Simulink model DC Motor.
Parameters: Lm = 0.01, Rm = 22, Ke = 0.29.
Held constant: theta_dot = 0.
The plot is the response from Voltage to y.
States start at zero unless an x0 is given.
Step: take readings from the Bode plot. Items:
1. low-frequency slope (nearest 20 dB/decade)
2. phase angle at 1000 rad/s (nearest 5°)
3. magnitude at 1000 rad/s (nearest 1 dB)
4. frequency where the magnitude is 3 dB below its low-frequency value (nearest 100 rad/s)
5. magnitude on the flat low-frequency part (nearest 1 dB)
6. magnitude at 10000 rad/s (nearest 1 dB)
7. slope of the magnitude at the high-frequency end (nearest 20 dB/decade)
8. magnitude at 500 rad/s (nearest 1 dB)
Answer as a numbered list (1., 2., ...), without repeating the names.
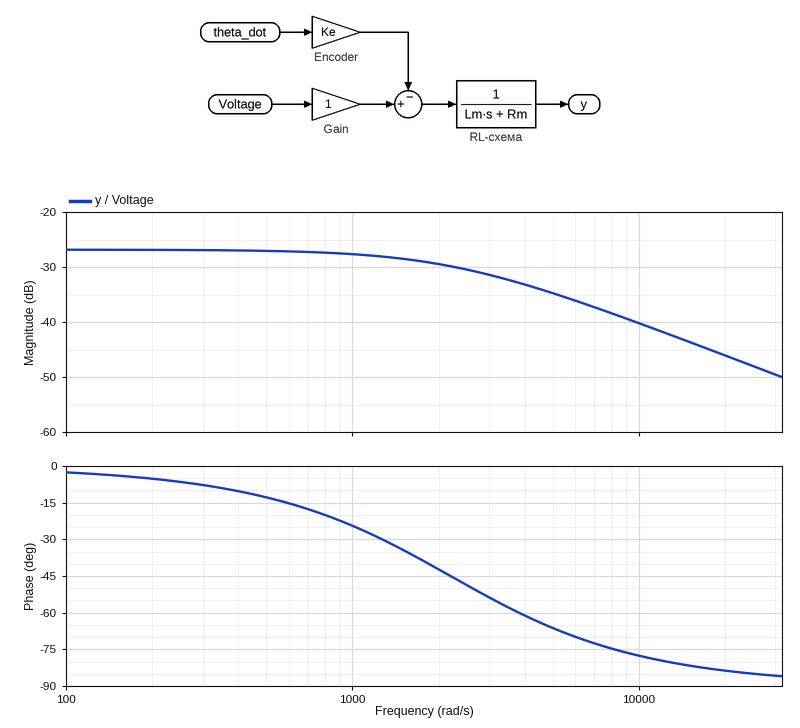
1. 0 dB/decade
2. -25°
3. -28 dB
4. 2200 rad/s
5. -27 dB
6. -40 dB
7. -20 dB/decade
8. -27 dB
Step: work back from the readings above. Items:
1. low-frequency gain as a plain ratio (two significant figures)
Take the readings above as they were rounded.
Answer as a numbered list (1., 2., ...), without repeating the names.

1. 0.045
